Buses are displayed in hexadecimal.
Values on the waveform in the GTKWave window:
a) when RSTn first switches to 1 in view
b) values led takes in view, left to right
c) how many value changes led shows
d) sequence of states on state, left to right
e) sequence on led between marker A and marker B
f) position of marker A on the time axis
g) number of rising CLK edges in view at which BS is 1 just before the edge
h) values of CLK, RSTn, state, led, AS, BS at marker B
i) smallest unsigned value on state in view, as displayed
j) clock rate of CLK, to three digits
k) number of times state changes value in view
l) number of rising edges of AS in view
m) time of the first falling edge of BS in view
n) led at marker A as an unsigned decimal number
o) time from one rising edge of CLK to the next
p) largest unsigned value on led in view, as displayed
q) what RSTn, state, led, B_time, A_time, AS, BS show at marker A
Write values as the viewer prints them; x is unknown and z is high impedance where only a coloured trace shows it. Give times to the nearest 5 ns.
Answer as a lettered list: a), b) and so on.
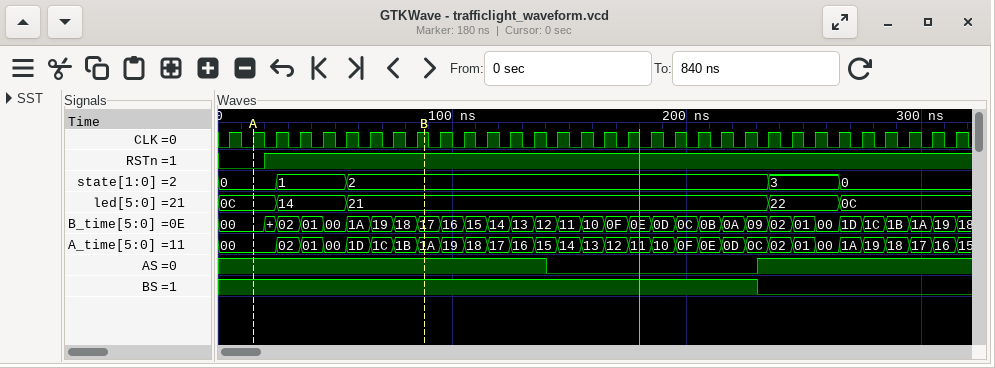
a) 20 ns
b) 0C, 14, 21, 22, 0C
c) 4
d) 0, 1, 2, 3, 0
e) 0C, 14, 21
f) 15 ns
g) 23
h) CLK=1, RSTn=1, state=2, led=21, AS=1, BS=1
i) 0
j) 100 MHz
k) 4
l) 1
m) 230 ns
n) 12
o) 10 ns
p) 22
q) RSTn=0, state=0, led=0C, B_time=00, A_time=00, AS=1, BS=1
